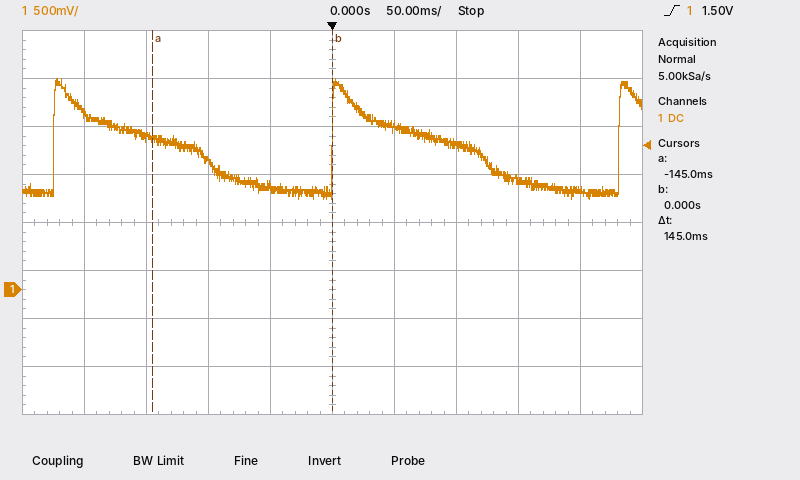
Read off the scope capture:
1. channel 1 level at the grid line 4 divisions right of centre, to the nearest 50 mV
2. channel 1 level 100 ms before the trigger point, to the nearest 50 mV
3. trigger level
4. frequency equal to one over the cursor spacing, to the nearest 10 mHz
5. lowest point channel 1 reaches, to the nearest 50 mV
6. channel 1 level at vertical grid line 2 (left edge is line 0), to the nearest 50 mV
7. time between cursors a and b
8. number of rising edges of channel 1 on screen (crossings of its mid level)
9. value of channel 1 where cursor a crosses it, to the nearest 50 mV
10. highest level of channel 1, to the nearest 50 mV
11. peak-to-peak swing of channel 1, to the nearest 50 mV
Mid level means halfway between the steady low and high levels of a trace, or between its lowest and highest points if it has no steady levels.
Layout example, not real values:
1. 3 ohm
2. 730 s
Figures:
1. 1.05 V
2. 1.35 V
3. 1.50 V
4. 6.90 Hz
5. 950 mV
6. 1.60 V
7. 145 ms
8. 3
9. 1.60 V
10. 2.20 V
11. 1.25 V
